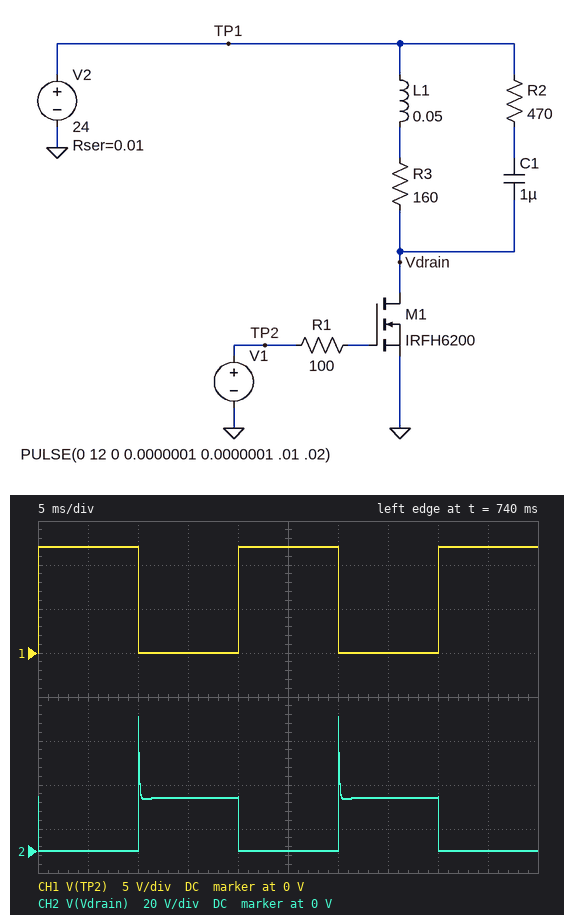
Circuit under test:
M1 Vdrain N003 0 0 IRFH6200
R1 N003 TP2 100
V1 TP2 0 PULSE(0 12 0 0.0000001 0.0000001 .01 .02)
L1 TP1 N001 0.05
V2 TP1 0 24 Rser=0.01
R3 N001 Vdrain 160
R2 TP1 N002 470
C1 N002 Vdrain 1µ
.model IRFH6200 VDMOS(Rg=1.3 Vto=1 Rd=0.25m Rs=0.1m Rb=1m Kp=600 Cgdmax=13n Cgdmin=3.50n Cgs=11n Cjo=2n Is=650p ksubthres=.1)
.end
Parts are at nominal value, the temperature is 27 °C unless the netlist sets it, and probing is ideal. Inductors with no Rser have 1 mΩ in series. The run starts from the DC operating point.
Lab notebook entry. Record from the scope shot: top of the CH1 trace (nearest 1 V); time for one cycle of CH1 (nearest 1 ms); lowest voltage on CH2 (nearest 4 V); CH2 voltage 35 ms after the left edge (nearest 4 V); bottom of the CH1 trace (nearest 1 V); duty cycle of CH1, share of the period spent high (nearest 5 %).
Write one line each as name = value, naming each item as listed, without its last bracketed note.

top of the CH1 trace = 12 V
time for one cycle of CH1 = 20 ms
lowest voltage on CH2 = 0 V
CH2 voltage 35 ms after the left edge = 24 V
bottom of the CH1 trace = 0 V
duty cycle of CH1, share of the period spent high = 50 %
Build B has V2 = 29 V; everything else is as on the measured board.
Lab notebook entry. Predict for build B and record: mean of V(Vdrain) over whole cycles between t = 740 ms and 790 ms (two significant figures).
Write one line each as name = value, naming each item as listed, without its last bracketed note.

mean of V(Vdrain) over whole cycles between t = 740 ms and 790 ms = 15 V
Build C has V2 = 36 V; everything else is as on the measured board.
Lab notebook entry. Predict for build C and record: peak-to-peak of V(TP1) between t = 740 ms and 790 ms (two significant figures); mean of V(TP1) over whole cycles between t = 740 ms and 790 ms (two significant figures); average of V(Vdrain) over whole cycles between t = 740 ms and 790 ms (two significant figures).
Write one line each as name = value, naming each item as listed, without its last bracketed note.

peak-to-peak of V(TP1) between t = 740 ms and 790 ms = 2.3 mV
mean of V(TP1) over whole cycles between t = 740 ms and 790 ms = 36 V
average of V(Vdrain) over whole cycles between t = 740 ms and 790 ms = 18 V
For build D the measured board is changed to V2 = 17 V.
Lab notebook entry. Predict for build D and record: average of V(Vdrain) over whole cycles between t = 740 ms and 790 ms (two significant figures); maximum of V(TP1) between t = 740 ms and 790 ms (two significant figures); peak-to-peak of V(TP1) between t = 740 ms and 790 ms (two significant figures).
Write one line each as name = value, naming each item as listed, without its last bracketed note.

average of V(Vdrain) over whole cycles between t = 740 ms and 790 ms = 8.6 V
maximum of V(TP1) between t = 740 ms and 790 ms = 17 V
peak-to-peak of V(TP1) between t = 740 ms and 790 ms = 1.1 mV
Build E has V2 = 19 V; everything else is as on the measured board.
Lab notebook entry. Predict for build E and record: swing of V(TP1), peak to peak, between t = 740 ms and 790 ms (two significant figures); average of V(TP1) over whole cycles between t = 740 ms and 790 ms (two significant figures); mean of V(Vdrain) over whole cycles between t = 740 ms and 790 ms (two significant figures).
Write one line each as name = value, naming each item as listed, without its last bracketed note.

swing of V(TP1), peak to peak, between t = 740 ms and 790 ms = 1.2 mV
average of V(TP1) over whole cycles between t = 740 ms and 790 ms = 19 V
mean of V(Vdrain) over whole cycles between t = 740 ms and 790 ms = 9.6 V
